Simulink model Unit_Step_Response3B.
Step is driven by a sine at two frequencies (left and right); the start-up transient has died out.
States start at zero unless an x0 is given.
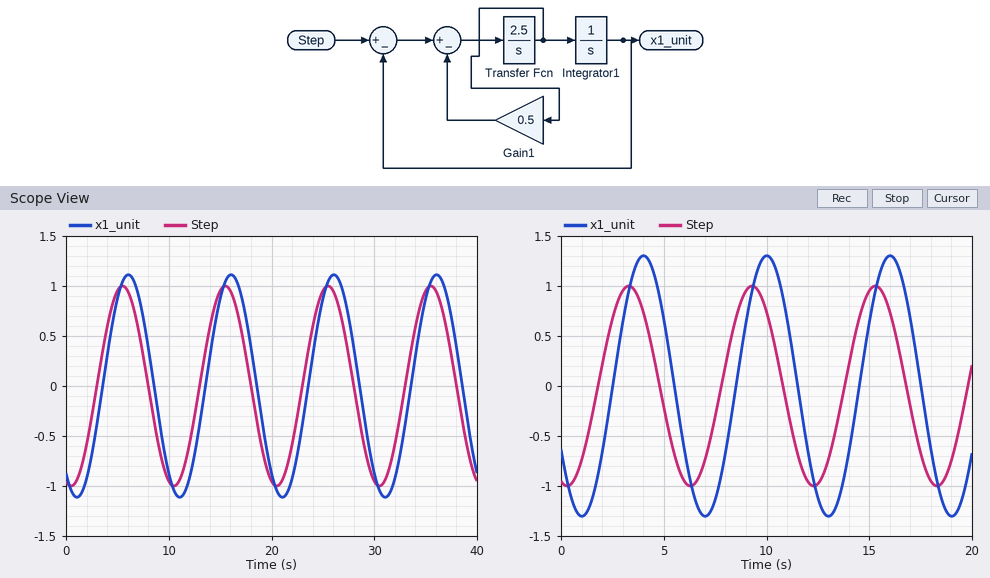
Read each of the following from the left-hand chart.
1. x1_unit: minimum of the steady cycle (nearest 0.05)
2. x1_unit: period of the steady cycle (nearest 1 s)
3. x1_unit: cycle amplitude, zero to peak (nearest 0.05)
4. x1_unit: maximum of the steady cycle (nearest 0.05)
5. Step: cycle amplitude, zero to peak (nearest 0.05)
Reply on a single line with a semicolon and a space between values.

-1.10; 10 s; 1.10; 1.10; 1.00
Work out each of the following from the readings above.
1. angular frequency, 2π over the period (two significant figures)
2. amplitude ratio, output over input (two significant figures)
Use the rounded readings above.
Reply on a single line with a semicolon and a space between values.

0.63 rad/s; 1.1
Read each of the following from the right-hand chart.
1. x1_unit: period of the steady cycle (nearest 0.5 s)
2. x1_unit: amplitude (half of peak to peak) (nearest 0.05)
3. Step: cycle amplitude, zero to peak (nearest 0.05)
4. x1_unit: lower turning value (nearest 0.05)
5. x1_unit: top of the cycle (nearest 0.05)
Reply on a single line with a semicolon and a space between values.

6.0 s; 1.30; 1.00; -1.30; 1.30
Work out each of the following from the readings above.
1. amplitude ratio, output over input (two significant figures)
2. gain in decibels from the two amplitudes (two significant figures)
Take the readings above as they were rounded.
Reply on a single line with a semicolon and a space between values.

1.3; 2.3 dB
